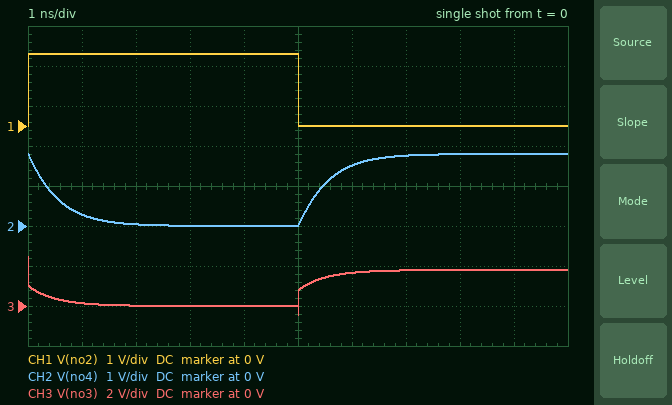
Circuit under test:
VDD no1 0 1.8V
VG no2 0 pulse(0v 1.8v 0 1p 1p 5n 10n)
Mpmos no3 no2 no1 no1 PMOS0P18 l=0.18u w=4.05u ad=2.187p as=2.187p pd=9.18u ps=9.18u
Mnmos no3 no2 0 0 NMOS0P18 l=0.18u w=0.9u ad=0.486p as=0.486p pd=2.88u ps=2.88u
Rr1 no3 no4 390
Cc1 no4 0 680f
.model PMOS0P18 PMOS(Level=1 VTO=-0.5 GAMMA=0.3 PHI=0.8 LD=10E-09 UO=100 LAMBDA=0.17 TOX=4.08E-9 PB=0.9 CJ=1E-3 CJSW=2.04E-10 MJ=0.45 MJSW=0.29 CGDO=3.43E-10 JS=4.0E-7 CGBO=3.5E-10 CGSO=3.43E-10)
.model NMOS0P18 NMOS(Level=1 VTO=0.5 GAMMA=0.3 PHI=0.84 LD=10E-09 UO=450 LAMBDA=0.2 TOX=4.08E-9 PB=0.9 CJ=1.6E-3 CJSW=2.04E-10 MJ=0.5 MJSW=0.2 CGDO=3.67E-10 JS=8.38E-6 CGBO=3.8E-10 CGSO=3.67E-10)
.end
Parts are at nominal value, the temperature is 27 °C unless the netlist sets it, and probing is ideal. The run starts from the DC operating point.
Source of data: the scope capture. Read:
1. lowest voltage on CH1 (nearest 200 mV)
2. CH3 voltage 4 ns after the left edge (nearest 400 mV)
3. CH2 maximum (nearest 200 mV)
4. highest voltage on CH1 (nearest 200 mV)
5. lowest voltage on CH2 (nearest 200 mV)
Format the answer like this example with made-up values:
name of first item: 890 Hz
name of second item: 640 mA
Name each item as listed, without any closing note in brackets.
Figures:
lowest voltage on CH1: 0 V
CH3 voltage 4 ns after the left edge: 0 V
CH2 maximum: 1.8 V
highest voltage on CH1: 1.8 V
lowest voltage on CH2: 0 V
